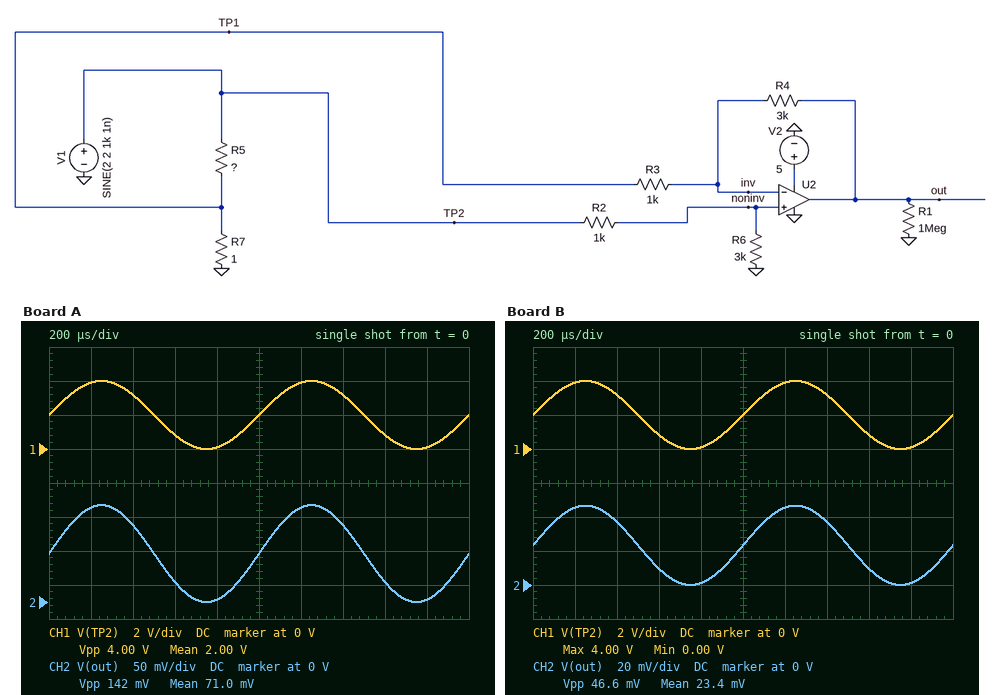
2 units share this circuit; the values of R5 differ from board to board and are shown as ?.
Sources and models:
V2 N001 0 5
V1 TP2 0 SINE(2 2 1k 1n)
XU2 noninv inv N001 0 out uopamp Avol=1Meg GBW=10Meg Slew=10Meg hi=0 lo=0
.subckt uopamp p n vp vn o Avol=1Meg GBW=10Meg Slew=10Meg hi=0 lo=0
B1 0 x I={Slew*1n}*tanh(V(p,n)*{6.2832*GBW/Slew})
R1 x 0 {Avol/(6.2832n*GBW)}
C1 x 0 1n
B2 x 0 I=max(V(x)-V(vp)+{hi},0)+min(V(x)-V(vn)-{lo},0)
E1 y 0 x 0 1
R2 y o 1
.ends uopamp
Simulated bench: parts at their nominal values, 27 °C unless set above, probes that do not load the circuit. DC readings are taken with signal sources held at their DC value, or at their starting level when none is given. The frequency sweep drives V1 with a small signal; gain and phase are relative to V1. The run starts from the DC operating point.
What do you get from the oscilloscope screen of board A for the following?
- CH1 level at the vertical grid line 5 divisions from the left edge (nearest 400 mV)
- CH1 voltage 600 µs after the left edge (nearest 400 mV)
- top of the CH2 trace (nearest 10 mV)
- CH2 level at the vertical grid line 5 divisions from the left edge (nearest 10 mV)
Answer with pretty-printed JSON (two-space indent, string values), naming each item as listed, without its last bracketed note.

{
  "CH1 level at the vertical grid line 5 divisions from the left edge": "2.0 V",
  "CH1 voltage 600 µs after the left edge": "800 mV",
  "top of the CH2 trace": "140 mV",
  "CH2 level at the vertical grid line 5 divisions from the left edge": "70 mV"
}
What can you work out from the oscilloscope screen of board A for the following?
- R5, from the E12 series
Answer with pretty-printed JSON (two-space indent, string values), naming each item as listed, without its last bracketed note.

{
  "R5, from the E12 series": "0.012 Ω"
}
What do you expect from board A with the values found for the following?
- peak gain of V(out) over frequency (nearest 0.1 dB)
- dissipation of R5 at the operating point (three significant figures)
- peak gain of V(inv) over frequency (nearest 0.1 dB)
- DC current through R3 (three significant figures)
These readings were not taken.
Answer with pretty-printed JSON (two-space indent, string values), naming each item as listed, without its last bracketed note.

{
  "peak gain of V(out) over frequency": "-29.0 dB",
  "dissipation of R5 at the operating point": "46.9 mW",
  "peak gain of V(inv) over frequency": "-2.5 dB",
  "DC current through R3": "476 µA"
}
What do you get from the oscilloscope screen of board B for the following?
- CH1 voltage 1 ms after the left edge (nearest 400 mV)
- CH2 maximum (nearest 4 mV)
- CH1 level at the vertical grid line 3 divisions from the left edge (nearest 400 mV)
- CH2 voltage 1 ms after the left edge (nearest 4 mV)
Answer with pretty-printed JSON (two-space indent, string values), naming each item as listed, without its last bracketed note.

{
  "CH1 voltage 1 ms after the left edge": "2.0 V",
  "CH2 maximum": "48 mV",
  "CH1 level at the vertical grid line 3 divisions from the left edge": "800 mV",
  "CH2 voltage 1 ms after the left edge": "24 mV"
}
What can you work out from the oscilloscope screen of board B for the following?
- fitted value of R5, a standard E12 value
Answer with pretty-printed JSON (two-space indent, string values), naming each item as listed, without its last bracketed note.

{
  "fitted value of R5, a standard E12 value": "3.9 mΩ"
}
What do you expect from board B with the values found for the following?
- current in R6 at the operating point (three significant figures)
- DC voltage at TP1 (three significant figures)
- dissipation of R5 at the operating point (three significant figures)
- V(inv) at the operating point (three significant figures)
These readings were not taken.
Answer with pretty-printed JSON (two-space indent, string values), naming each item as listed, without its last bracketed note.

{
  "current in R6 at the operating point": "500 µA",
  "DC voltage at TP1": "1.99 V",
  "dissipation of R5 at the operating point": "15.5 mW",
  "V(inv) at the operating point": "1.50 V"
}
